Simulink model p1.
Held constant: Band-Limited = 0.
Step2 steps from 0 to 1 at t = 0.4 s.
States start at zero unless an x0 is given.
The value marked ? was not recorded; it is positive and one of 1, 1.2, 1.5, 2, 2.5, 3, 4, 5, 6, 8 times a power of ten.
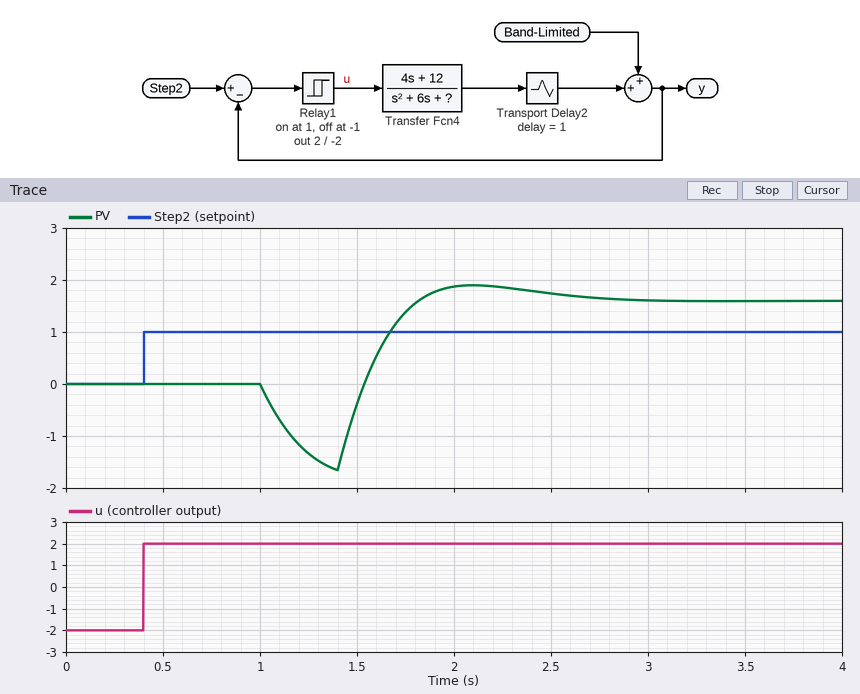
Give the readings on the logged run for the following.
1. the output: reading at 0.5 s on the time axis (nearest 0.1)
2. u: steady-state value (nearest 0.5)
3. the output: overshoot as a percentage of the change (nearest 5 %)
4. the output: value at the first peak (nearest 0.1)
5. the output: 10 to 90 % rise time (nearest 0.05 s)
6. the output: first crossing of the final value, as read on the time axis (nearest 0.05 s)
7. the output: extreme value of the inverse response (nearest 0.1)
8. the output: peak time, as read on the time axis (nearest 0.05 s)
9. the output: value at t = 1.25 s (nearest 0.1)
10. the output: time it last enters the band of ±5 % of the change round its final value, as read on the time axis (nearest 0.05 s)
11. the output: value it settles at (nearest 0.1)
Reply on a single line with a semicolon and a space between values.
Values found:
0.0; 2.0; 20 %; 1.9; 0.20 s; 1.80 s; -1.7; 2.10 s; -1.3; 2.65 s; 1.6
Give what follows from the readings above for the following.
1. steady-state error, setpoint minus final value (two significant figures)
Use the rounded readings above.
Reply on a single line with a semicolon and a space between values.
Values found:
-0.60
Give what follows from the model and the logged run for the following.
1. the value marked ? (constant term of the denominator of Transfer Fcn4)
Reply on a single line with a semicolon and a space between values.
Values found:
15
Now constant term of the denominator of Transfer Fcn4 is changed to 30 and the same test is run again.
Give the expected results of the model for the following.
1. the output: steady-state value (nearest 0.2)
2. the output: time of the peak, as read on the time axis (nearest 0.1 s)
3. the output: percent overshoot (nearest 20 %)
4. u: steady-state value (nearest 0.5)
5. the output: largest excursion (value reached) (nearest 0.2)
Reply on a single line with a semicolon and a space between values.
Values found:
0.8; 1.8 s; 100 %; 2.0; 1.6
